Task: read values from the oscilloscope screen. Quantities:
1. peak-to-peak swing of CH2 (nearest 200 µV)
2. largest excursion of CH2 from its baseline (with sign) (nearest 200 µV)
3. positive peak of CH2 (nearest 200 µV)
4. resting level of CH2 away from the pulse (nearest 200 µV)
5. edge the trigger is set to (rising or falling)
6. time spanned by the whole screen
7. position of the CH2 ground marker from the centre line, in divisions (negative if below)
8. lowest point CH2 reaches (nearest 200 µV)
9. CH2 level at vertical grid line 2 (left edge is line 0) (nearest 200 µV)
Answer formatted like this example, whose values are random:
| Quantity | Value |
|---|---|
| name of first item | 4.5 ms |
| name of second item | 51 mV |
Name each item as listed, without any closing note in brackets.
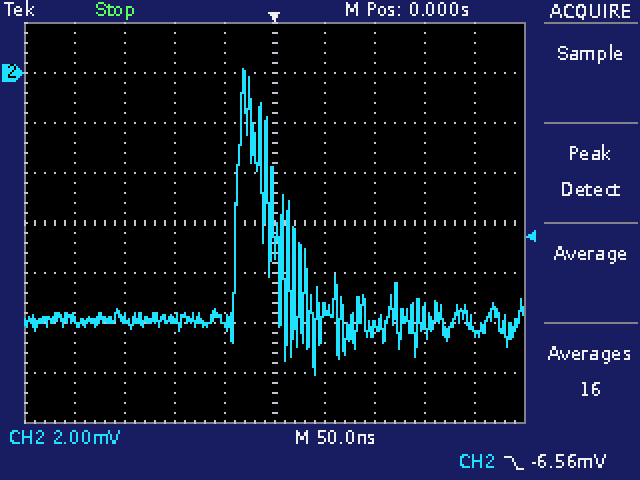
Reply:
| Quantity | Value |
|---|---|
| peak-to-peak swing of CH2 | 12.2 mV |
| largest excursion of CH2 from its baseline (with sign) | +10.0 mV |
| positive peak of CH2 | 200 µV |
| resting level of CH2 away from the pulse | -9.8 mV |
| edge the trigger is set to | falling |
| time spanned by the whole screen | 500 ns |
| position of the CH2 ground marker from the centre line, in divisions | +3.0 div |
| lowest point CH2 reaches | -12.0 mV |
| CH2 level at vertical grid line 2 (left edge is line 0) | -9.8 mV |
